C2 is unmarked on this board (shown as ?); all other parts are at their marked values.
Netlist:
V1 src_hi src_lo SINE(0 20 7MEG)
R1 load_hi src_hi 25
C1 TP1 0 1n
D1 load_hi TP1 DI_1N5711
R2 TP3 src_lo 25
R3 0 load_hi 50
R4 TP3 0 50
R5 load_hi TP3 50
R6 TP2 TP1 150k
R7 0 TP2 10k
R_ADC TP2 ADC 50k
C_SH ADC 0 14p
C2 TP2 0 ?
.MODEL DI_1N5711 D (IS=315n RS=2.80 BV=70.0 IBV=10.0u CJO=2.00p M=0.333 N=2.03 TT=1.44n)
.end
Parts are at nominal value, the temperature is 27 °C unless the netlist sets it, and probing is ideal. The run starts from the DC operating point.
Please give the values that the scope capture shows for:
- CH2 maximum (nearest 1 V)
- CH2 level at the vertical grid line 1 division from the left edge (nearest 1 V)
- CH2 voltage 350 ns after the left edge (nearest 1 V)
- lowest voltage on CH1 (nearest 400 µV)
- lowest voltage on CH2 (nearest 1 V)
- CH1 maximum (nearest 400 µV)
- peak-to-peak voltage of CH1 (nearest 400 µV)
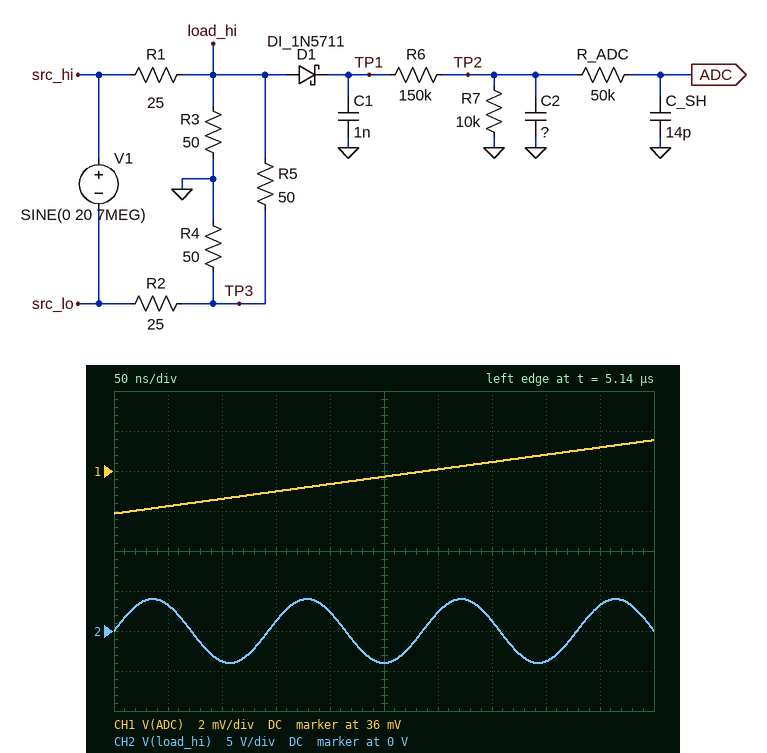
4 V
3 V
1 V
34.0 mV
-4 V
37.6 mV
3.6 mV
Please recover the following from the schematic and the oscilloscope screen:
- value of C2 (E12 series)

2.7 nF
